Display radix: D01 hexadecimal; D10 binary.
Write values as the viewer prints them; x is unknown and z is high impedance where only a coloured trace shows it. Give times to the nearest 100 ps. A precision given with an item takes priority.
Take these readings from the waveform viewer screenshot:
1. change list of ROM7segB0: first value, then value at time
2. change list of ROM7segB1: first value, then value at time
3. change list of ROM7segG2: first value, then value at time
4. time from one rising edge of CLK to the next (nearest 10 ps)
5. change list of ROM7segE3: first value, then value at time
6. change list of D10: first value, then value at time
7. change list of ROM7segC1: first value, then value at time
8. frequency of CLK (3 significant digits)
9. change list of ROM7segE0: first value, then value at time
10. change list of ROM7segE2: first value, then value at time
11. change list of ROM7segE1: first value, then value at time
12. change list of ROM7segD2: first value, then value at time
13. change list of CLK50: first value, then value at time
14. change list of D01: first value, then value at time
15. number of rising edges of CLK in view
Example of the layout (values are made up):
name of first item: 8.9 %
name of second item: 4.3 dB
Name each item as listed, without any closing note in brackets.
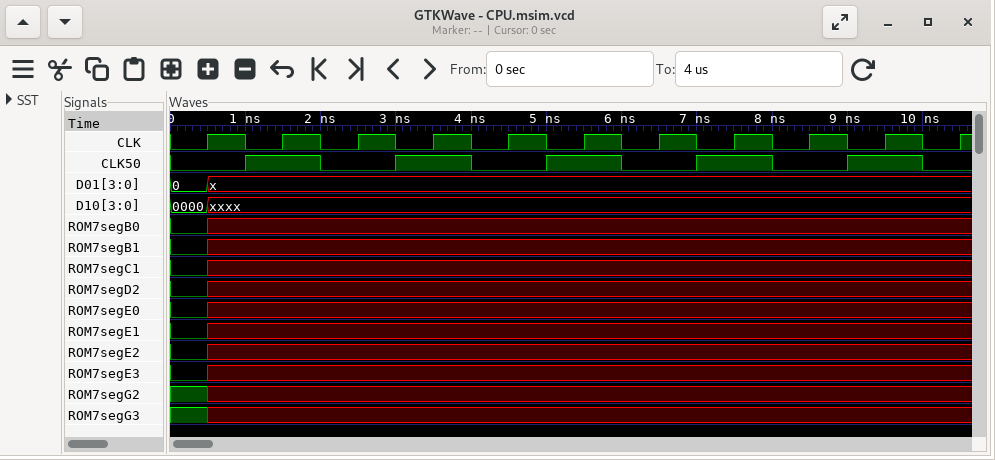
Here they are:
change list of ROM7segB0: first value, then value at time: 0, x at 500 ps
change list of ROM7segB1: first value, then value at time: 0, x at 500 ps
change list of ROM7segG2: first value, then value at time: 1, x at 500 ps
time from one rising edge of CLK to the next: 1000 ps
change list of ROM7segE3: first value, then value at time: 0, x at 500 ps
change list of D10: first value, then value at time: 0000, xxxx at 500 ps
change list of ROM7segC1: first value, then value at time: 0, x at 500 ps
frequency of CLK: 1.00 GHz
change list of ROM7segE0: first value, then value at time: 0, x at 500 ps
change list of ROM7segE2: first value, then value at time: 0, x at 500 ps
change list of ROM7segE1: first value, then value at time: 0, x at 500 ps
change list of ROM7segD2: first value, then value at time: 0, x at 500 ps
change list of CLK50: first value, then value at time: 0, 1 at 1000 ps, 0 at 2000 ps, 1 at 3000 ps, 0 at 4000 ps, 1 at 5000 ps, 0 at 6000 ps, 1 at 7000 ps, 0 at 8000 ps, 1 at 9000 ps, 0 at 10000 ps
change list of D01: first value, then value at time: 0, x at 500 ps
number of rising edges of CLK in view: 11
